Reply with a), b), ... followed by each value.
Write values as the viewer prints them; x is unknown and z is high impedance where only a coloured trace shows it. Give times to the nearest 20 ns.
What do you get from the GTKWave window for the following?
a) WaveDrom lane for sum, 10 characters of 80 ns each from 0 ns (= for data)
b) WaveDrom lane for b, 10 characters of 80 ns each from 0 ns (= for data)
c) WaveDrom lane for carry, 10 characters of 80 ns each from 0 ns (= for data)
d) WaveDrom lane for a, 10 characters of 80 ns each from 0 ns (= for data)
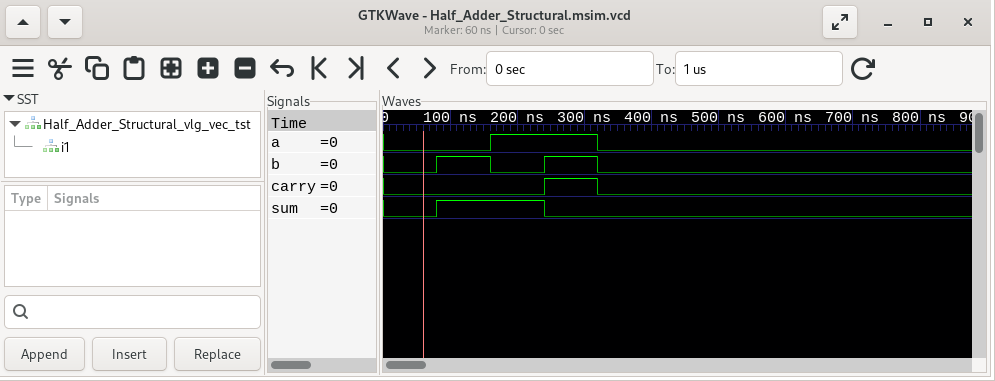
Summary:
a) {name: 'sum', wave: '01.0......'}
b) {name: 'b', wave: '01010.....'}
c) {name: 'carry', wave: '0..10.....'}
d) {name: 'a', wave: '0.1.0.....'}
